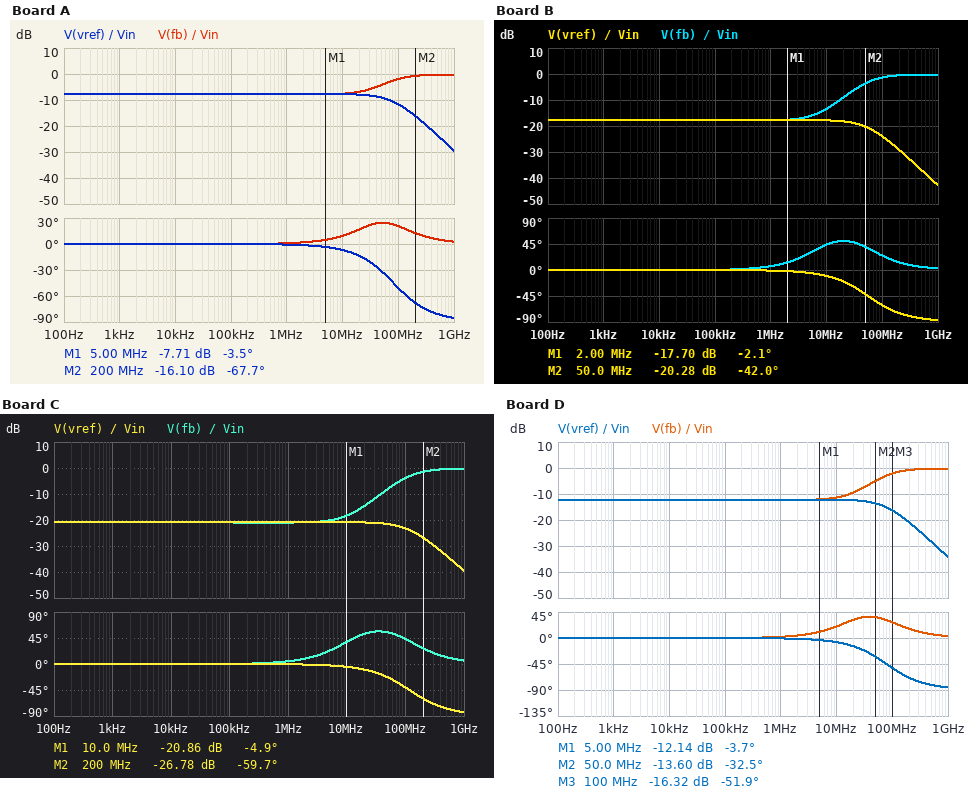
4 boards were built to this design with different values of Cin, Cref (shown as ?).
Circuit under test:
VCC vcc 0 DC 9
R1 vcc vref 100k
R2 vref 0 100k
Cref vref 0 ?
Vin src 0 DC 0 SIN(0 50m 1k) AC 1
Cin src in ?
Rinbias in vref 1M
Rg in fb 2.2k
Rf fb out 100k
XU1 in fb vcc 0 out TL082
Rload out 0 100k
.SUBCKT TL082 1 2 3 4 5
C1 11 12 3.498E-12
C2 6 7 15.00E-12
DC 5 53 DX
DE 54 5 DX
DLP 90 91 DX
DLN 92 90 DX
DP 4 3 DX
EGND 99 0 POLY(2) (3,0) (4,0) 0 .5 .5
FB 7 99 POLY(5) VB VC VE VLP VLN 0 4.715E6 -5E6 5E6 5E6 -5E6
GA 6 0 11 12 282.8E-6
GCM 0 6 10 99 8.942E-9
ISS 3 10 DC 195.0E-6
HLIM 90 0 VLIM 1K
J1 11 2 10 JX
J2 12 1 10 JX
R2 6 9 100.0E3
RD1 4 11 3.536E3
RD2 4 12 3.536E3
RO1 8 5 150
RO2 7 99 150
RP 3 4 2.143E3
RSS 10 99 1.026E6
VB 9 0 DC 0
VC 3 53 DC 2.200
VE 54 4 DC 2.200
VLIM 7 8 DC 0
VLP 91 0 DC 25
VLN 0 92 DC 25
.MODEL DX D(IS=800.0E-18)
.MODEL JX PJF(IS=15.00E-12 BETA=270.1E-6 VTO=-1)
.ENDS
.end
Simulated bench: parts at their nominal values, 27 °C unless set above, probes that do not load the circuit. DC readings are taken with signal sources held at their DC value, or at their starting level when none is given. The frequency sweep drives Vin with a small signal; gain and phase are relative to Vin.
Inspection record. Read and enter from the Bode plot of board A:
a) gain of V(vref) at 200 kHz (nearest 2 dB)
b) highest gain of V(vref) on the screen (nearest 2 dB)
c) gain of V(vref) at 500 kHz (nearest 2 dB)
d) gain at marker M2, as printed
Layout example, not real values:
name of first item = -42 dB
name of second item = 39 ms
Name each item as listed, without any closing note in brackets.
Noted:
gain of V(vref) at 200 kHz = -8 dB
highest gain of V(vref) on the screen = -8 dB
gain of V(vref) at 500 kHz = -8 dB
gain at marker M2, as printed = -16.10 dB
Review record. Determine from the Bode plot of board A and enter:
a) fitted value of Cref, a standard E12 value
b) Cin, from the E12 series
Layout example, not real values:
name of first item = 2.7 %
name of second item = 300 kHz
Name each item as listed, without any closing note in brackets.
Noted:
fitted value of Cref, a standard E12 value = 4.7 µF
Cin, from the E12 series = 3.3 µF
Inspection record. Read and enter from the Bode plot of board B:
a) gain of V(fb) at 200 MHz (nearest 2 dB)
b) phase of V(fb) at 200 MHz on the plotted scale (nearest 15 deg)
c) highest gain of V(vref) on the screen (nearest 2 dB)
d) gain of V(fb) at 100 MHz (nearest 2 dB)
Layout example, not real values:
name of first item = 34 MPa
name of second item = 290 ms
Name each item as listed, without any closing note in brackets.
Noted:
gain of V(fb) at 200 MHz = 0 dB
phase of V(fb) at 200 MHz on the plotted scale = 15 deg
highest gain of V(vref) on the screen = -18 dB
gain of V(fb) at 100 MHz = -2 dB
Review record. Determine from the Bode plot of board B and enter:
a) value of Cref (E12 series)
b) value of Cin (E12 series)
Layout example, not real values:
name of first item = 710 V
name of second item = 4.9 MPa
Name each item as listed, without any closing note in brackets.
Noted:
value of Cref = 22 µF
value of Cin = 3.3 µF
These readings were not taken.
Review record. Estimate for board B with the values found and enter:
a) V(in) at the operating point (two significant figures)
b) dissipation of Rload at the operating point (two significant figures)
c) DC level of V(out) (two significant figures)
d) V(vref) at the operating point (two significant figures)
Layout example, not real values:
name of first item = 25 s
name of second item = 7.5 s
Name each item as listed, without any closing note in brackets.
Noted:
V(in) at the operating point = 4.5 V
dissipation of Rload at the operating point = 200 µW
DC level of V(out) = 4.5 V
V(vref) at the operating point = 4.5 V
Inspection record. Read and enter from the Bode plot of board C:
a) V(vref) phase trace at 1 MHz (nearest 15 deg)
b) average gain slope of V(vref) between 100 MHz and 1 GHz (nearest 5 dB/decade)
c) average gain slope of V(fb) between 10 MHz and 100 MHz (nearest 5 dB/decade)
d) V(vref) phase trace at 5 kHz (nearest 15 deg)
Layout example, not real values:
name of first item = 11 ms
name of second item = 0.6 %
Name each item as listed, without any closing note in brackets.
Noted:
V(vref) phase trace at 1 MHz = 0 deg
average gain slope of V(vref) between 100 MHz and 1 GHz = -15 dB/decade
average gain slope of V(fb) between 10 MHz and 100 MHz = 15 dB/decade
V(vref) phase trace at 5 kHz = 0 deg
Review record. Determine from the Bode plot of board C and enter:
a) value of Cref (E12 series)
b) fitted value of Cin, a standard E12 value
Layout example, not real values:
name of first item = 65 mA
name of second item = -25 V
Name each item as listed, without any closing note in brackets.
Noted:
value of Cref = 15 µF
fitted value of Cin, a standard E12 value = 1.5 µF
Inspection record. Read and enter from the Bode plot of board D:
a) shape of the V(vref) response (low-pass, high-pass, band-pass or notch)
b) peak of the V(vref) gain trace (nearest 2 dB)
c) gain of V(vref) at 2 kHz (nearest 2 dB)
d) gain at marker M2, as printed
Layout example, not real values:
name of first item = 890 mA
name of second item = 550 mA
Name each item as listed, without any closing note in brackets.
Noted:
shape of the V(vref) response = low-pass
peak of the V(vref) gain trace = -12 dB
gain of V(vref) at 2 kHz = -12 dB
gain at marker M2, as printed = -13.60 dB
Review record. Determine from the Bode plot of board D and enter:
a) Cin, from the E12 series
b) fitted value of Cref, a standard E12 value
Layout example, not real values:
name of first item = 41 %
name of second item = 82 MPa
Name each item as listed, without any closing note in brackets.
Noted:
Cin, from the E12 series = 2.7 µF
fitted value of Cref, a standard E12 value = 8.2 µF
